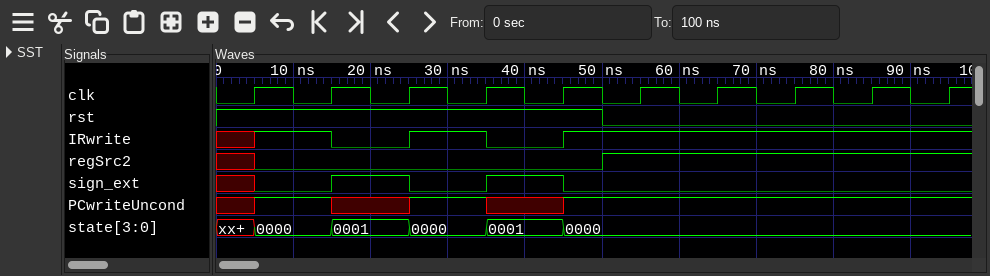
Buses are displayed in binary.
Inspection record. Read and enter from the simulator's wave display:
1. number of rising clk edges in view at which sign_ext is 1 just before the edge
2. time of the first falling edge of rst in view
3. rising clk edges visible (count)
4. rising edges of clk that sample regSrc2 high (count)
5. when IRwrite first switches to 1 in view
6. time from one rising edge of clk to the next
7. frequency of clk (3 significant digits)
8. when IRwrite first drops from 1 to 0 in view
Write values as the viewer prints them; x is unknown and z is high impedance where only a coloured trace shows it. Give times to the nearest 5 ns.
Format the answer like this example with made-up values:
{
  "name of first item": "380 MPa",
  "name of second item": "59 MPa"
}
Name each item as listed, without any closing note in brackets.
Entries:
{
  "number of rising clk edges in view at which sign_ext is 1 just before the edge": "2",
  "time of the first falling edge of rst in view": "50 ns",
  "rising clk edges visible": "10",
  "rising edges of clk that sample regSrc2 high": "5",
  "when IRwrite first switches to 1 in view": "5 ns",
  "time from one rising edge of clk to the next": "10 ns",
  "frequency of clk": "100 MHz",
  "when IRwrite first drops from 1 to 0 in view": "15 ns"
}
